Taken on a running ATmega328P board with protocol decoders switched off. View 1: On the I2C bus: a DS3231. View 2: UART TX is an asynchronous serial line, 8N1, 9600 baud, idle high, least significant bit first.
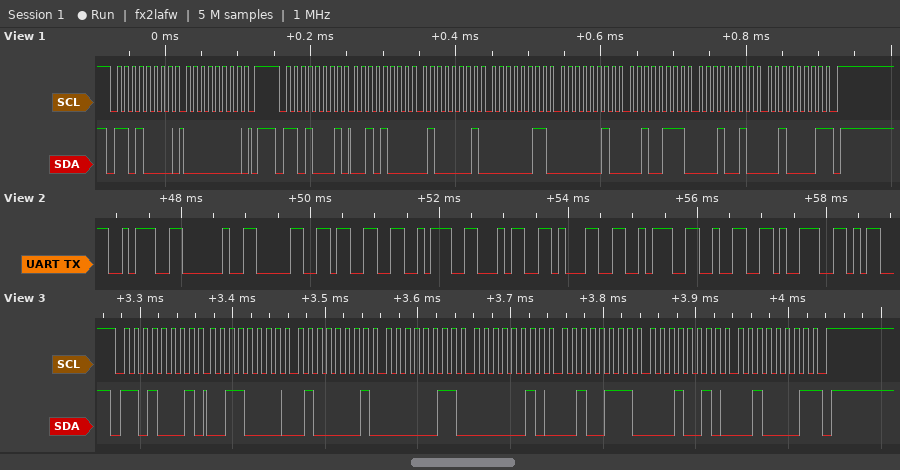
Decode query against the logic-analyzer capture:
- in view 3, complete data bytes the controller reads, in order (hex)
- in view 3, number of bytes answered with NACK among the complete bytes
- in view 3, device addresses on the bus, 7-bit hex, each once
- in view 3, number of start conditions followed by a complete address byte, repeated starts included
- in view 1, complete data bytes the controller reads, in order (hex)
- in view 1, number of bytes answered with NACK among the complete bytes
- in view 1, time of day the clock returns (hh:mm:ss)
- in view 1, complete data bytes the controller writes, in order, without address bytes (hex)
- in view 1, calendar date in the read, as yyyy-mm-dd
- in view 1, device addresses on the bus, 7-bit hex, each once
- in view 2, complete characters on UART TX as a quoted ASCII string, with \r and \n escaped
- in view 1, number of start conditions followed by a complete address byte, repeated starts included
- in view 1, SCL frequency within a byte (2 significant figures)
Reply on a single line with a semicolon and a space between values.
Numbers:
30 41 03 02 27 12 21; 1; 0x68; 1; 28 41 03 02 27 12 21; 1; 03:41:28; 00; 2021-12-27; 0x68; ": 03:41:29"; 2; 100 kHz
